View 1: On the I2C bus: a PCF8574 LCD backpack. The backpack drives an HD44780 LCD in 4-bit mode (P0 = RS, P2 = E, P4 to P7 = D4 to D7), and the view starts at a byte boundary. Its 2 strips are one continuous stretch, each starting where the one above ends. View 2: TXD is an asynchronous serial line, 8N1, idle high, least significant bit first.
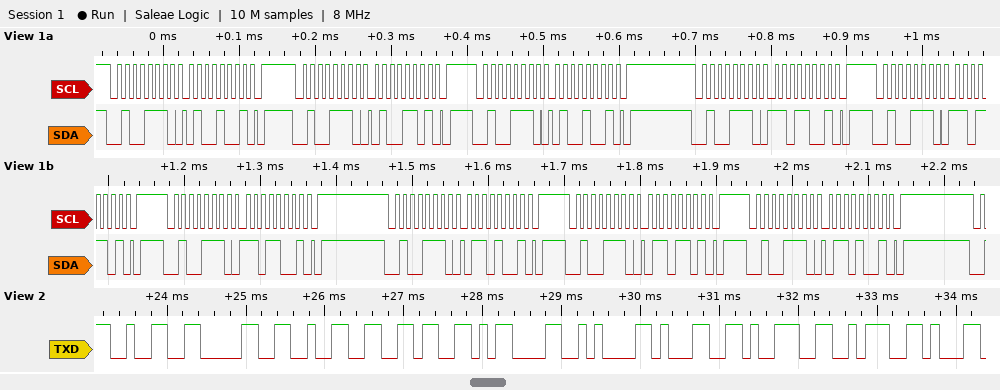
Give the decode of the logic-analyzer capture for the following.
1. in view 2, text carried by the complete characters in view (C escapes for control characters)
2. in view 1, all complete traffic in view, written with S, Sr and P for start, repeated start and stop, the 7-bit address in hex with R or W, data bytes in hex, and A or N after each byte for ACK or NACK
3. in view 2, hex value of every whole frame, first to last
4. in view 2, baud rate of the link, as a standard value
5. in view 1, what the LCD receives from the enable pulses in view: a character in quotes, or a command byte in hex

"2026\r\n19:"
S 27W A 49 A P S 27W A 4D A P S 27W A 49 A P S 27W A D9 A P S 27W A DD A P S 27W A D9 A P S 27W A 69 A P S 27W A 6D A P S 27W A 69 A P
32 30 32 36 0D 0A 31 39 3A
9600 baud
'M'
